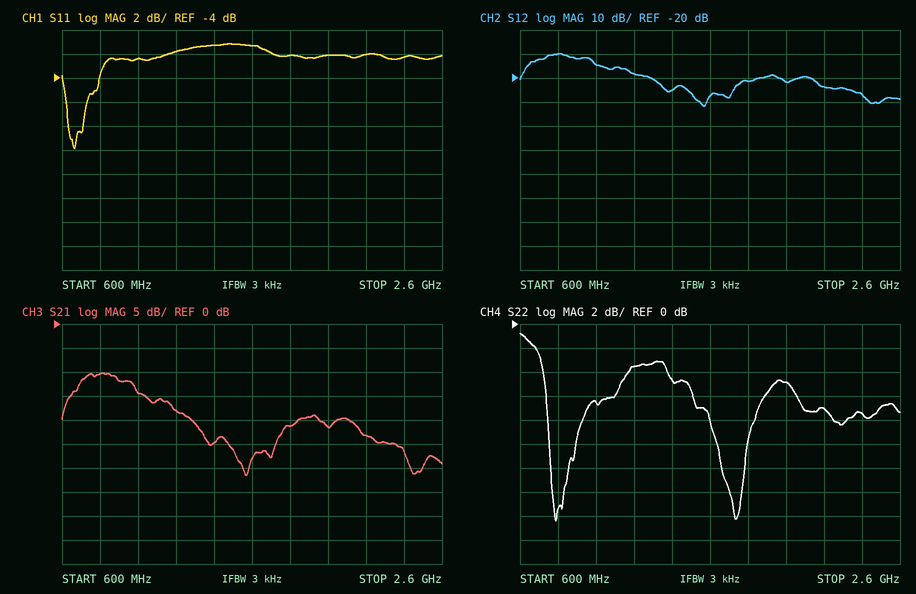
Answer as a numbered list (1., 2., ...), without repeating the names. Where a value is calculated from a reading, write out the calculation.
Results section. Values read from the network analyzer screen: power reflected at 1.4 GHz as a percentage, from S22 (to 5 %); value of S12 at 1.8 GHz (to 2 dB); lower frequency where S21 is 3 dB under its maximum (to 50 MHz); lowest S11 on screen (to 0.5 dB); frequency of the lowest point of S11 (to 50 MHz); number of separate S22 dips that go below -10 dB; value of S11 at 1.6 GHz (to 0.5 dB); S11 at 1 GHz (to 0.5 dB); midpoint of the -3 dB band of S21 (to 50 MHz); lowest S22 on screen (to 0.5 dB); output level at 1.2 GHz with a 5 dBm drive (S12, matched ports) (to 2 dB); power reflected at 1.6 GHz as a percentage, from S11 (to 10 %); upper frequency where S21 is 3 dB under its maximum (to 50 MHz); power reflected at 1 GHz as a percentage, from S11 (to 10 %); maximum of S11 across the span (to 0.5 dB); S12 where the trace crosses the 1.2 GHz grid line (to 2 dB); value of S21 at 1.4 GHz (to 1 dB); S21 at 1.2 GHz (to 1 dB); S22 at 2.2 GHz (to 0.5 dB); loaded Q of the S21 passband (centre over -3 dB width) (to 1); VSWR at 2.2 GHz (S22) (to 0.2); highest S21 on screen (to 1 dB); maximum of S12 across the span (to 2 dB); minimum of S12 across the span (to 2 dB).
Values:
1. 10^(-4.5/10) ≈ 35 %
2. -22 dB
3. 700 MHz
4. -10.0 dB
5. 650 MHz
6. 2
7. -1.5 dB
8. -2.5 dB
9. 850 MHz
10. -16.5 dB
11. 5 dBm + (-18 dB) = -14 dBm
12. 10^(-1.5/10) ≈ 70.8 %, so 70 % to the nearest 10 %
13. 1.00 GHz
14. 10^(-2.5/10) ≈ 56.2 %, so 60 % to the nearest 10 %
15. -1.0 dB
16. -18 dB
17. -25 dB
18. -18 dB
19. -7.0 dB
20. 850 MHz / 300 MHz ≈ 3
21. |Γ| = 10^(-7/20) = 0.4467; VSWR = (1 + 0.4467)/(1 − 0.4467) ≈ 2.6
22. -10 dB
23. -10 dB
24. -32 dB
